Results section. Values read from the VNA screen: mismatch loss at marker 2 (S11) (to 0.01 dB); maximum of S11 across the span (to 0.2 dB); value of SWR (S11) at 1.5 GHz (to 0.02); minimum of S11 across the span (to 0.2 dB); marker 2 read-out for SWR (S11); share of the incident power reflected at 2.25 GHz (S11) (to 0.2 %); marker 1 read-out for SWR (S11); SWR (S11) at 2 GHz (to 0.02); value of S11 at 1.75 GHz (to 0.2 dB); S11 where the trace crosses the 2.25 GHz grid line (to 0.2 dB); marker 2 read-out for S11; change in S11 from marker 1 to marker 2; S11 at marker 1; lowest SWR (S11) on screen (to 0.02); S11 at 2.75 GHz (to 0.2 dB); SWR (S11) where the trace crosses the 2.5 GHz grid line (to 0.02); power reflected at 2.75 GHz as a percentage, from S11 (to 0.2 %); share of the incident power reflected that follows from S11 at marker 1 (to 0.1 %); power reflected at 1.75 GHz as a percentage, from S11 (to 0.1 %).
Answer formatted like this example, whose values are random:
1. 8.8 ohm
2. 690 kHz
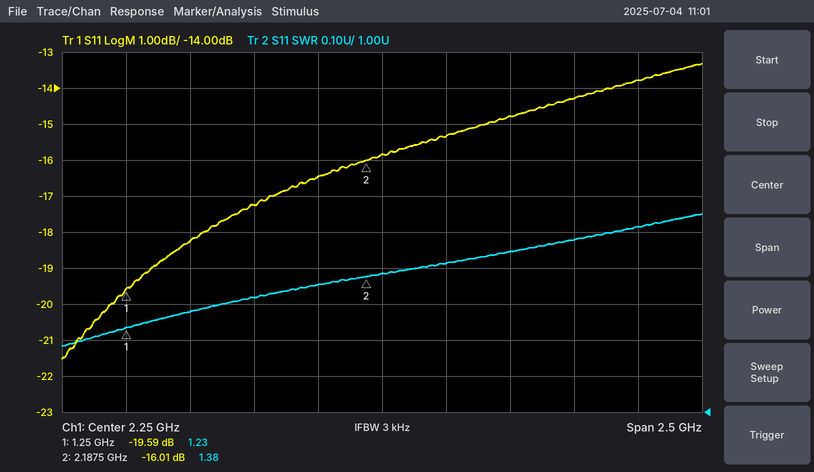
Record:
1. 0.11 dB
2. -13.4 dB
3. 1.28
4. -21.6 dB
5. 1.38
6. 2.6 %
7. 1.23
8. 1.36
9. -17.2 dB
10. -15.8 dB
11. -16.01 dB
12. 3.58 dB
13. -19.59 dB
14. 1.18
15. -14.8 dB
16. 1.42
17. 3.4 %
18. 1.1 %
19. 1.9 %
